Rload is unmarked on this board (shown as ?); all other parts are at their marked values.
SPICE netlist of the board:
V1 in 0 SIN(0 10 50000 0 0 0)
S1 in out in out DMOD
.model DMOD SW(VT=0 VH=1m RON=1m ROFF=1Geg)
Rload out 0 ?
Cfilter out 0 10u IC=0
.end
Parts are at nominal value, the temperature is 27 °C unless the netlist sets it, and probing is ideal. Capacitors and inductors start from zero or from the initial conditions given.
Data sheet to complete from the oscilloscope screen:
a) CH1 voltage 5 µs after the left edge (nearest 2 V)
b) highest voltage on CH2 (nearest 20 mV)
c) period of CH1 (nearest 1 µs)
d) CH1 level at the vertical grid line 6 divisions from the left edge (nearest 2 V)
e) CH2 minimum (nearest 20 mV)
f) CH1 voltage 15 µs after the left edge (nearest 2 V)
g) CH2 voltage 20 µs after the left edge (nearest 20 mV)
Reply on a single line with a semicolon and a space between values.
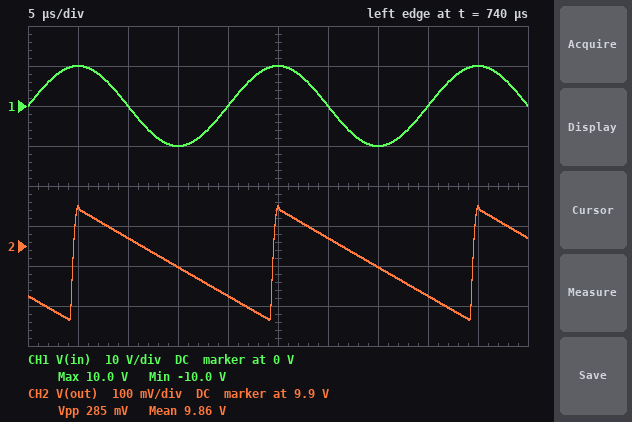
10 V; 10.00 V; 20 µs; 0 V; 9.72 V; -10 V; 9.78 V
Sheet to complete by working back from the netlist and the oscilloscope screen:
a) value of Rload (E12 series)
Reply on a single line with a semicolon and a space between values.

68 Ω
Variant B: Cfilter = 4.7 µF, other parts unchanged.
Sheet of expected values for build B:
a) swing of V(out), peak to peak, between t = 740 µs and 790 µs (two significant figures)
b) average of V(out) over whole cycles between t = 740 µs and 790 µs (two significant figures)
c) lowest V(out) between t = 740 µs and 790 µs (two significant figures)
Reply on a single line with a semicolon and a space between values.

590 mV; 9.7 V; 9.4 V
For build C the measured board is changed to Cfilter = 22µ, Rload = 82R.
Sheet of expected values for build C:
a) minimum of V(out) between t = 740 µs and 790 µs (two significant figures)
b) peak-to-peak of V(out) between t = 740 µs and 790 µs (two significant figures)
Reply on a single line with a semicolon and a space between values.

9.9 V; 110 mV
